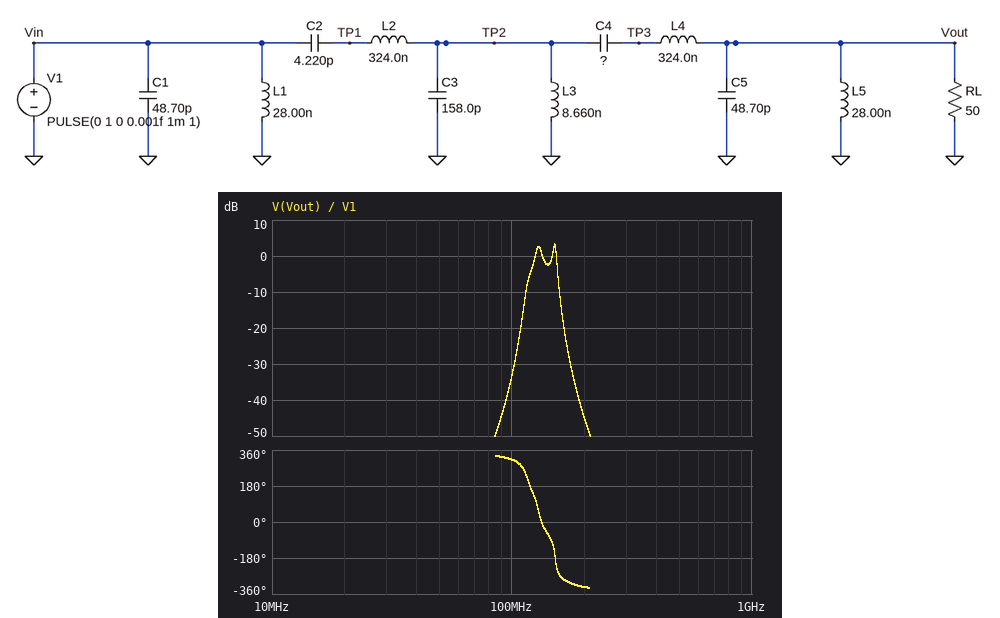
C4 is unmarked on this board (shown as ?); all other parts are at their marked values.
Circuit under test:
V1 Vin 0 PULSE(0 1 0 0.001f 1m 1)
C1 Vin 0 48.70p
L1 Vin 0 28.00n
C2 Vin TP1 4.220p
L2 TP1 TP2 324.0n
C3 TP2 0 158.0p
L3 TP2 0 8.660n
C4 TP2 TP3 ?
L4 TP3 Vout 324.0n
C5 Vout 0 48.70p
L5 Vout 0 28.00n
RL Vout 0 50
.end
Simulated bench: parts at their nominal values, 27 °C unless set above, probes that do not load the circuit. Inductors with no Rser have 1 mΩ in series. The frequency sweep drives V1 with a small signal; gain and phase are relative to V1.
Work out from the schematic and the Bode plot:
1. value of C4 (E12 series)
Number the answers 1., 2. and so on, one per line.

1. 4.7 pF
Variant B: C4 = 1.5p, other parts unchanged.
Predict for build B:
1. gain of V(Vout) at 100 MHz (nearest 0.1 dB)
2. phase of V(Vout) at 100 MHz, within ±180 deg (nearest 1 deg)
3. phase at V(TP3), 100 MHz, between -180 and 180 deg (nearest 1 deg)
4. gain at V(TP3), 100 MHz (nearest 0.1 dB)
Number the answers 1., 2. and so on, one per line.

1. -51.4 dB
2. -39 deg
3. -6 deg
4. -33.8 dB
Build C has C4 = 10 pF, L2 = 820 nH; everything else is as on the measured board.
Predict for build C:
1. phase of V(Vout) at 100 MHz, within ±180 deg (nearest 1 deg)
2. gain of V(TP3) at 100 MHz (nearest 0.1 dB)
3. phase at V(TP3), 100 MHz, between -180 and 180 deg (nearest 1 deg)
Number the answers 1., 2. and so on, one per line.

1. -24 deg
2. -13.1 dB
3. 8 deg
